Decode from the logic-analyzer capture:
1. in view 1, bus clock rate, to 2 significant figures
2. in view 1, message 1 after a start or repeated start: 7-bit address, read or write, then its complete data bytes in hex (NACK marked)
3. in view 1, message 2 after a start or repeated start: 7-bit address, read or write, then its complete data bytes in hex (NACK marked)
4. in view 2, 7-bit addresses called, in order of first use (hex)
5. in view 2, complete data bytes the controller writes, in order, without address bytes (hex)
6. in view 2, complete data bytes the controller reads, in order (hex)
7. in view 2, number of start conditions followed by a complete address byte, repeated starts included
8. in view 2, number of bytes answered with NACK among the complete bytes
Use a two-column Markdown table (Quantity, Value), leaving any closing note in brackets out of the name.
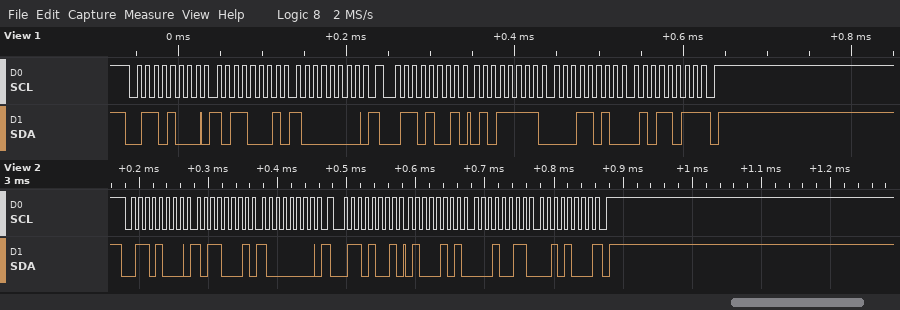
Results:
| Quantity | Value |
|---|---|
| in view 1, bus clock rate, to 2 significant figures | 100 kHz |
| in view 1, message 1 after a start or repeated start: 7-bit address, read or write, then its complete data bytes in hex | 0x34 write: B1 80 |
| in view 1, message 2 after a start or repeated start: 7-bit address, read or write, then its complete data bytes in hex | 0x34 read: 5F 1A 5B NACK |
| in view 2, 7-bit addresses called, in order of first use | 0x34 |
| in view 2, complete data bytes the controller writes, in order, without address bytes | B1 80 |
| in view 2, complete data bytes the controller reads, in order | 45 13 28 |
| in view 2, number of start conditions followed by a complete address byte, repeated starts included | 2 |
| in view 2, number of bytes answered with NACK among the complete bytes | 1 |
